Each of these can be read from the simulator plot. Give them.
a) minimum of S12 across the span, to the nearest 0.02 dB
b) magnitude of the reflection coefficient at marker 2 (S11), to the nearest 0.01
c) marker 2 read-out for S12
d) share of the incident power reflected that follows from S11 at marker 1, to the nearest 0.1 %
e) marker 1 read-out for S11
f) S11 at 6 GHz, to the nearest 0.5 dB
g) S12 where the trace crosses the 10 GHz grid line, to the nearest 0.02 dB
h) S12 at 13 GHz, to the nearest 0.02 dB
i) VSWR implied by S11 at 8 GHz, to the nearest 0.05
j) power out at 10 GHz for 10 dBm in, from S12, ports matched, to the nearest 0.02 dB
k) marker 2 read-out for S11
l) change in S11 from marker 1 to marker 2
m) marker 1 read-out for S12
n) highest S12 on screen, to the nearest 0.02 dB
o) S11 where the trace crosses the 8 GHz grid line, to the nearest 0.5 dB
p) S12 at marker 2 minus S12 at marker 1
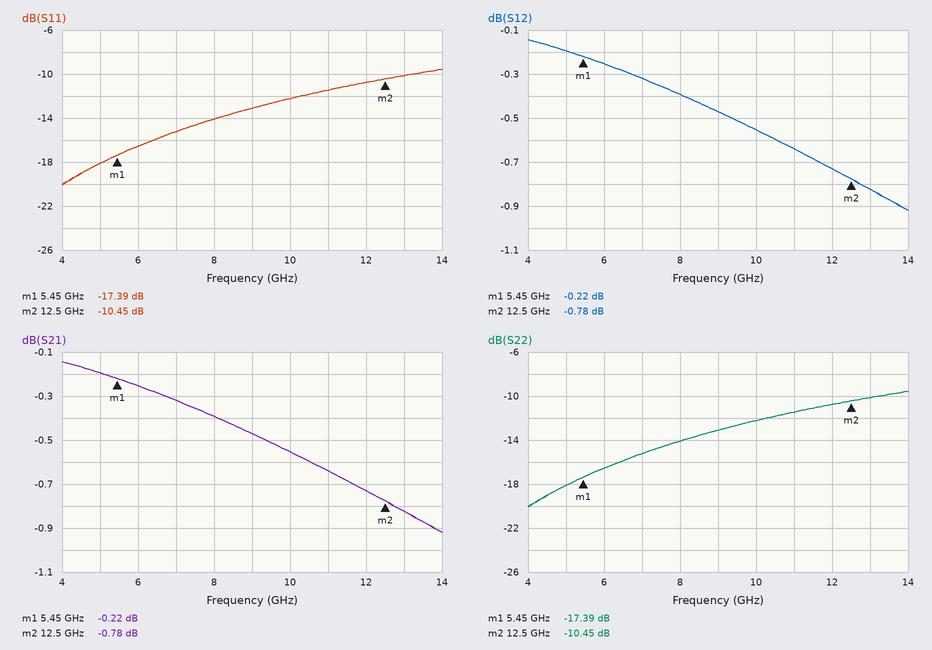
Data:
-0.92 dB
0.30
-0.78 dB
1.8 %
-17.39 dB
-16.5 dB
-0.56 dB
-0.82 dB
1.50
9.44 dBm
-10.45 dB
6.94 dB
-0.22 dB
-0.14 dB
-14.0 dB
-0.56 dB
